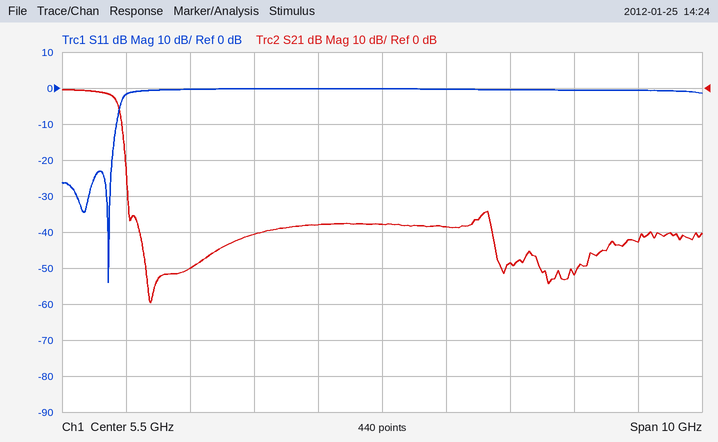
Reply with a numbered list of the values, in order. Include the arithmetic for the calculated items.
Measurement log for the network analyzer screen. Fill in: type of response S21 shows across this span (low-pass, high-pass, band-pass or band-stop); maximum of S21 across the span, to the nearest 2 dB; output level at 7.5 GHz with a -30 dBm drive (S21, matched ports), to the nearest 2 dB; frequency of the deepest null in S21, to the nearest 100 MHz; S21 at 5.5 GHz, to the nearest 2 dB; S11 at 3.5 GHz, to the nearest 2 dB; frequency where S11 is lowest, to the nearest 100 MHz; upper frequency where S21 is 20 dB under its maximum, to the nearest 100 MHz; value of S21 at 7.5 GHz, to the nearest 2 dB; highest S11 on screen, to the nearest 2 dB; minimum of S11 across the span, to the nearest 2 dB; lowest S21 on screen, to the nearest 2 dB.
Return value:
1. low-pass
2. 0 dB
3. -30 dBm + (-48 dB) = -78 dBm
4. 1.9 GHz
5. -38 dB
6. 0 dB
7. 1.2 GHz
8. 1.5 GHz
9. -48 dB
10. 0 dB
11. -54 dB
12. -60 dB
